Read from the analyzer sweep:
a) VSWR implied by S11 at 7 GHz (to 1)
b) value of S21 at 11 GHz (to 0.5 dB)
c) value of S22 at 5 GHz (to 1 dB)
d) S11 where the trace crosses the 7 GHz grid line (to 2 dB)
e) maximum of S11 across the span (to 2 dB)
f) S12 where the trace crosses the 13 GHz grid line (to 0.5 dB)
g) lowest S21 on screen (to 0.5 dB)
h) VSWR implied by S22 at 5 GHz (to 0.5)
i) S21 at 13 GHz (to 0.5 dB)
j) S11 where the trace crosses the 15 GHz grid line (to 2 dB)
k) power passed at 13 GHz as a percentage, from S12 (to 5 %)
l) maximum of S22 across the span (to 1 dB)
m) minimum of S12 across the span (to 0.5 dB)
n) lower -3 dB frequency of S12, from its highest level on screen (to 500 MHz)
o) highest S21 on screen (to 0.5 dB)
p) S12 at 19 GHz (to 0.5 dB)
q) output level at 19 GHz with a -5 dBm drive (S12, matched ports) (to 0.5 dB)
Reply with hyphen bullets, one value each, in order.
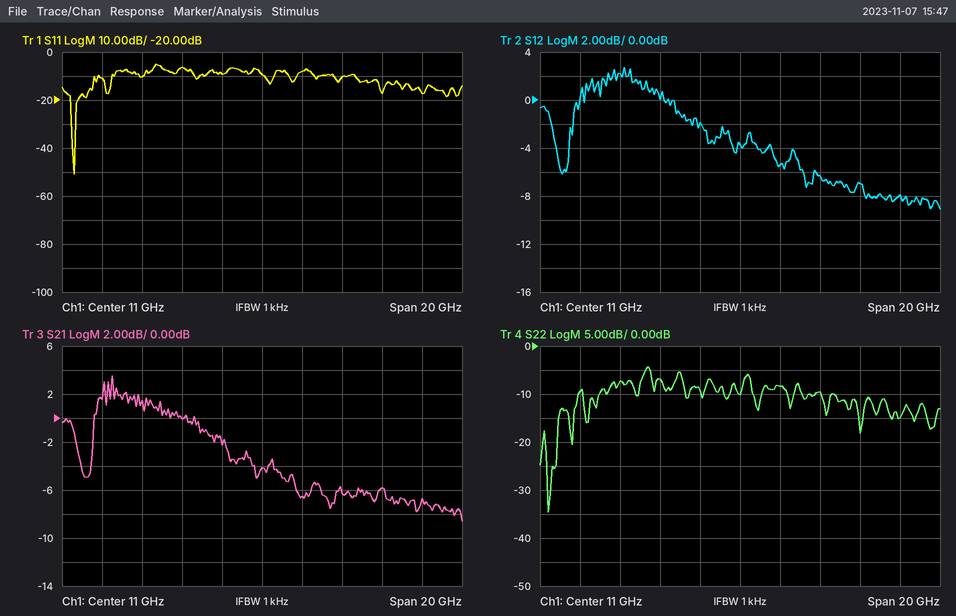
- 3
- -4.0 dB
- -7 dB
- -6 dB
- -6 dB
- -5.5 dB
- -8.5 dB
- 2.5
- -6.5 dB
- -10 dB
- 30 %
- -4 dB
- -9.0 dB
- 3.0 GHz
- 3.5 dB
- -8.0 dB
- -13.0 dBm
